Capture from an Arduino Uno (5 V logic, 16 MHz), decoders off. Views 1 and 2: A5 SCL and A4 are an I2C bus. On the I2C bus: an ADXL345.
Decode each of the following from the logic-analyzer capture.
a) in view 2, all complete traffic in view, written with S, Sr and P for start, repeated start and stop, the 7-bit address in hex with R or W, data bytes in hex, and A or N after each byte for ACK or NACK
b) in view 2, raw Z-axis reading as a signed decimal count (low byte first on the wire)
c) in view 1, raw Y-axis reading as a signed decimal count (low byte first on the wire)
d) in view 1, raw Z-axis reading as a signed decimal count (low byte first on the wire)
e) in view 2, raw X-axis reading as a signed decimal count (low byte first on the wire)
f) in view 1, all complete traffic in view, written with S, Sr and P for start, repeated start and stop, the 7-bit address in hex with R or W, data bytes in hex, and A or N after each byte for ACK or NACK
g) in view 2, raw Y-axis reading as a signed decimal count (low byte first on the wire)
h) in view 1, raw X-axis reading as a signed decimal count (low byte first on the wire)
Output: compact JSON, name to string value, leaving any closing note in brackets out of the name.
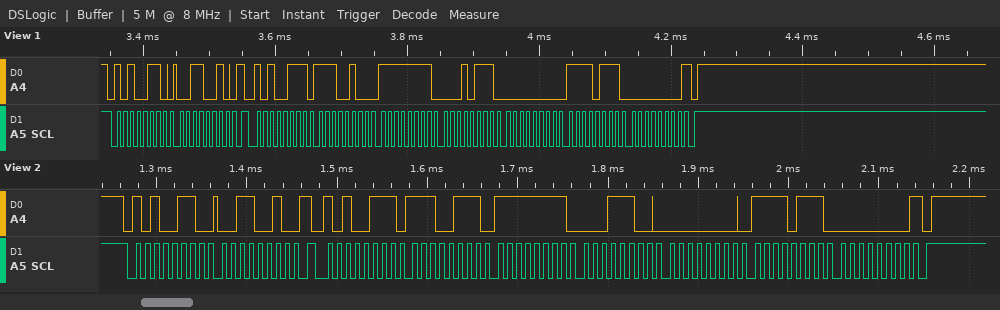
{"in view 2, all complete traffic in view, written with S, Sr and P for start, repeated start and stop, the 7-bit address in hex with R or W, data bytes in hex, and A or N after each byte for ACK or NACK": "S 53W A 32 A Sr 53R A E7 A FF A 1C A 00 A F7 A 00 N P", "in view 2, raw Z-axis reading as a signed decimal count": "247", "in view 1, raw Y-axis reading as a signed decimal count": "23", "in view 1, raw Z-axis reading as a signed decimal count": "247", "in view 2, raw X-axis reading as a signed decimal count": "-25", "in view 1, all complete traffic in view, written with S, Sr and P for start, repeated start and stop, the 7-bit address in hex with R or W, data bytes in hex, and A or N after each byte for ACK or NACK": "S 53W A 32 A Sr 53R A E4 A FF A 17 A 00 A F7 A 00 N P", "in view 2, raw Y-axis reading as a signed decimal count": "28", "in view 1, raw X-axis reading as a signed decimal count": "-28"}
